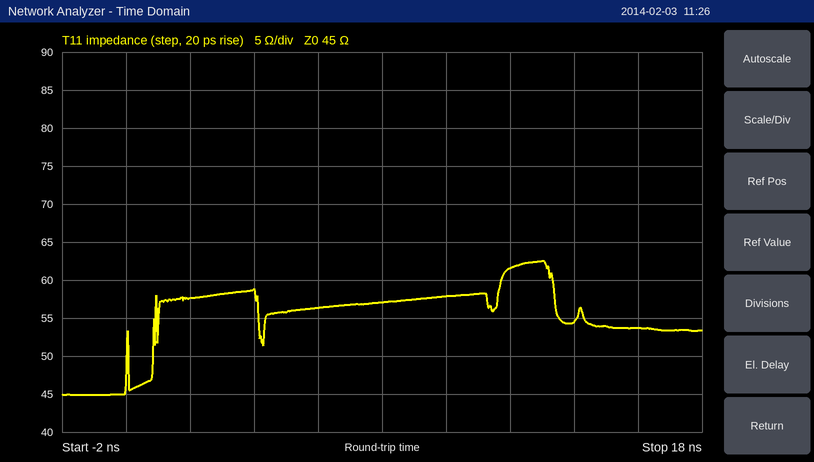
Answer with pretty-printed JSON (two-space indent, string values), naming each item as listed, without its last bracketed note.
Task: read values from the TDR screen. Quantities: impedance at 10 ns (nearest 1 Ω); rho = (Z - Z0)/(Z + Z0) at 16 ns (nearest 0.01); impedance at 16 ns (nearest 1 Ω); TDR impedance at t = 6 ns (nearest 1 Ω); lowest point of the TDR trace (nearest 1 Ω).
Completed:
{
  "impedance at 10 ns": "58 Ω",
  "rho = (Z - Z0)/(Z + Z0) at 16 ns": "+0.09",
  "impedance at 16 ns": "54 Ω",
  "TDR impedance at t = 6 ns": "56 Ω",
  "lowest point of the TDR trace": "45 Ω"
}
